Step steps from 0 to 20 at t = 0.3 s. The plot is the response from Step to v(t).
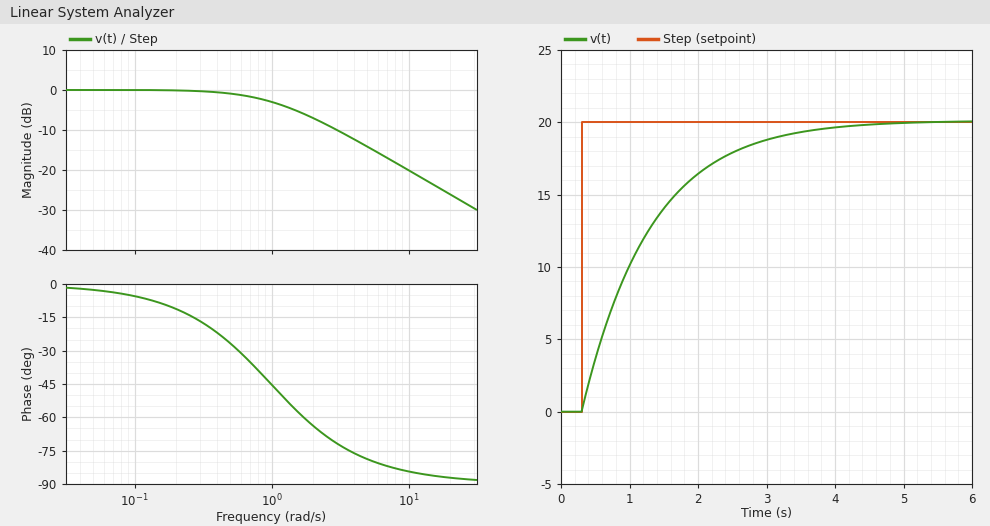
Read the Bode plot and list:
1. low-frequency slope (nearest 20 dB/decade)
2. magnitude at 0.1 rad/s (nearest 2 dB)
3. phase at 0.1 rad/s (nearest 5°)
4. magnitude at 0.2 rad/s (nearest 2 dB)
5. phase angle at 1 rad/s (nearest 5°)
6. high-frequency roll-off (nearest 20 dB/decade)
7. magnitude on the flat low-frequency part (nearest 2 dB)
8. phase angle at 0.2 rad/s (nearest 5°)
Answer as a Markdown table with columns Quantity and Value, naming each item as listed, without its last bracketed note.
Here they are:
| Quantity | Value |
|---|---|
| low-frequency slope | 0 dB/decade |
| magnitude at 0.1 rad/s | 0 dB |
| phase at 0.1 rad/s | -5° |
| magnitude at 0.2 rad/s | 0 dB |
| phase angle at 1 rad/s | -45° |
| high-frequency roll-off | -20 dB/decade |
| magnitude on the flat low-frequency part | 0 dB |
| phase angle at 0.2 rad/s | -10° |
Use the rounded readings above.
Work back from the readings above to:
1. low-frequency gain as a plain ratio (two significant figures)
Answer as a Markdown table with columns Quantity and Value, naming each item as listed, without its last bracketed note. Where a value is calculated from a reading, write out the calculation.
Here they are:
| Quantity | Value |
|---|---|
| low-frequency gain as a plain ratio | 10^(0 / 20) = 1.0 |
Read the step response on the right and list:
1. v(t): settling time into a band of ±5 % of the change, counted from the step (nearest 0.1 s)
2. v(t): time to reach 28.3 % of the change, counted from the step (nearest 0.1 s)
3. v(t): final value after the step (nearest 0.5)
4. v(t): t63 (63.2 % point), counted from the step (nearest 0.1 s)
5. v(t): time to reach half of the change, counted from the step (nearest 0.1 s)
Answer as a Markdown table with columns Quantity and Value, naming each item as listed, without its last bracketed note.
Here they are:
| Quantity | Value |
|---|---|
| v(t): settling time into a band of ±5 % of the change, counted from the step | 2.9 s |
| v(t): time to reach 28.3 % of the change, counted from the step | 0.3 s |
| v(t): final value after the step | 20.0 |
| v(t): t63 (63.2 % point), counted from the step | 1.0 s |
| v(t): time to reach half of the change, counted from the step | 0.7 s |
